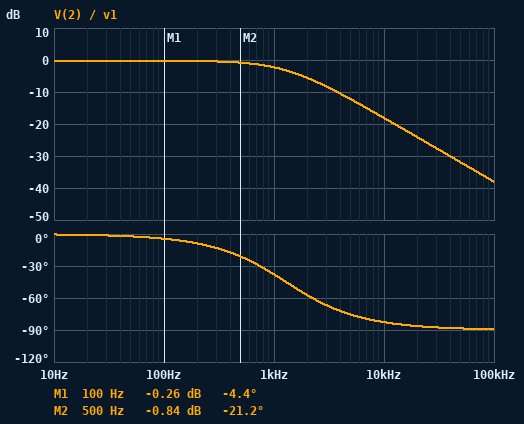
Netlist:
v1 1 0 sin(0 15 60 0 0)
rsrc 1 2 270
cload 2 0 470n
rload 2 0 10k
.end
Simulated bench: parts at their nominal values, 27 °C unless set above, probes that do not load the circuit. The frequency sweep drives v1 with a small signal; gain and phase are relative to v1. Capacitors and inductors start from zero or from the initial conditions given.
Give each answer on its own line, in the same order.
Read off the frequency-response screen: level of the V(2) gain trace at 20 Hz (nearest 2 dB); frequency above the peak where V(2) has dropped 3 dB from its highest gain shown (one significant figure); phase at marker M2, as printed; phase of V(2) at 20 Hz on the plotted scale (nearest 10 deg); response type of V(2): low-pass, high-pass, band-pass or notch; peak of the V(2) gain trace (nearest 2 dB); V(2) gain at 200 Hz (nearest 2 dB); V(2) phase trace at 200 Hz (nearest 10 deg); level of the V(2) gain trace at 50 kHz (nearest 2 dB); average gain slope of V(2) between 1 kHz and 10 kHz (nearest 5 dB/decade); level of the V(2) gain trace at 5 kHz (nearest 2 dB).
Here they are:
0 dB
1 kHz
-21.2 deg
0 deg
low-pass
0 dB
0 dB
-10 deg
-32 dB
-15 dB/decade
-12 dB
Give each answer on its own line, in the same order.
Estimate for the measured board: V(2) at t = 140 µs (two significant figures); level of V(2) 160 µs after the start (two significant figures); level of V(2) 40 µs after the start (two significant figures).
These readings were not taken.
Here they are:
310 mV
390 mV
32 mV
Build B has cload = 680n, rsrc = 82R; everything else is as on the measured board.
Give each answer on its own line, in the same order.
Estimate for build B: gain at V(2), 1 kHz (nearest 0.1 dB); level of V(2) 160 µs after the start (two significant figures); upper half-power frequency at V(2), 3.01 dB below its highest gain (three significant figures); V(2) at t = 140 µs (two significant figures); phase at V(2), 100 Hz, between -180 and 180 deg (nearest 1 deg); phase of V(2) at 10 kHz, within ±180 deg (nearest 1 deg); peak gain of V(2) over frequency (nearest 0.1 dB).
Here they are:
-0.6 dB
600 mV
2.88 kHz
500 mV
-2 deg
-74 deg
-0.1 dB
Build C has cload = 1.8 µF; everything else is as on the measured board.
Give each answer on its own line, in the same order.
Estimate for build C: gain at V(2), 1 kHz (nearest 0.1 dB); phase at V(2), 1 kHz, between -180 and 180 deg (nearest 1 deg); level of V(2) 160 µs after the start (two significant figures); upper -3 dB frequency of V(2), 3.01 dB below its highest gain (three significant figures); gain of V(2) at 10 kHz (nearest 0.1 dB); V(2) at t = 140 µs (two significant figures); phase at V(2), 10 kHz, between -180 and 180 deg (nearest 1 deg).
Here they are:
-10.2 dB
-71 deg
130 mV
336 Hz
-29.7 dB
100 mV
-88 deg
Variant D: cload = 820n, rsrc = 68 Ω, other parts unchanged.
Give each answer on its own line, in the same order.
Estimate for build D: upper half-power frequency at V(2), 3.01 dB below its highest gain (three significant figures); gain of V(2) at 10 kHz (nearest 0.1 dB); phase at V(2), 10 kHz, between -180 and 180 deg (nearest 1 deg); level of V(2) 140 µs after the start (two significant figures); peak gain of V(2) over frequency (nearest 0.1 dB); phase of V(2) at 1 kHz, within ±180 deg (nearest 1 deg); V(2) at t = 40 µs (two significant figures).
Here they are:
2.87 kHz
-11.2 dB
-74 deg
500 mV
-0.1 dB
-19 deg
65 mV
